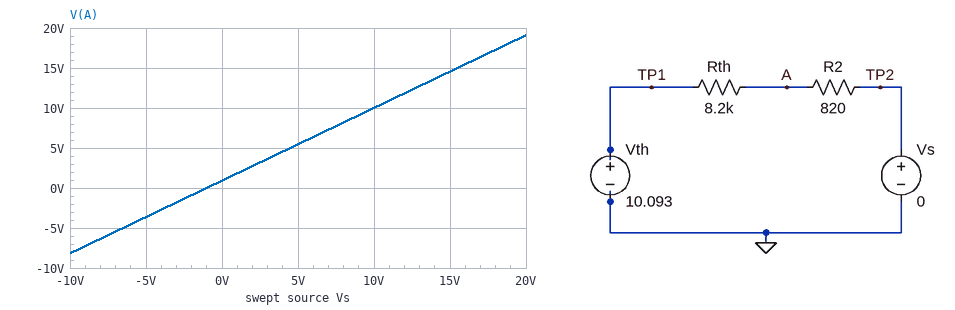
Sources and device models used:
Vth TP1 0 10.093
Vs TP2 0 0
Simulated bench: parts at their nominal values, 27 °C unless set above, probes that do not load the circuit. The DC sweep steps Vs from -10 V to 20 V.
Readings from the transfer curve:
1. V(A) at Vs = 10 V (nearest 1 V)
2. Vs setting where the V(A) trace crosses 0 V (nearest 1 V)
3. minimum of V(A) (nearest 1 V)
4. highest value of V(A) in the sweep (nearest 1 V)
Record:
10 V
-1 V
-8 V
19 V
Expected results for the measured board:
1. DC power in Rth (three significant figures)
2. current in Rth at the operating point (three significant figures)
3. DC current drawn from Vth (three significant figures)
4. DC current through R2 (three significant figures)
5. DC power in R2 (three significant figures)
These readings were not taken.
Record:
10.3 mW
1.12 mA
1.12 mA
1.12 mA
1.03 mW
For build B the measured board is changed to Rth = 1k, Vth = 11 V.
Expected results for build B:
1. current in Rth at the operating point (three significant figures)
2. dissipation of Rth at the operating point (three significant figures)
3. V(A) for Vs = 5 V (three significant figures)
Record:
6.04 mA
36.5 mW
7.70 V
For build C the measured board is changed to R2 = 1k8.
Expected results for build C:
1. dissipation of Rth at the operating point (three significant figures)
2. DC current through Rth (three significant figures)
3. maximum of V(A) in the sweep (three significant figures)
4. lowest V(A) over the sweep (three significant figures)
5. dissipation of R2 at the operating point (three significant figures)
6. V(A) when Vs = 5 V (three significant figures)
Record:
8.35 mW
1.01 mA
18.2 V
-6.38 V
1.83 mW
5.92 V
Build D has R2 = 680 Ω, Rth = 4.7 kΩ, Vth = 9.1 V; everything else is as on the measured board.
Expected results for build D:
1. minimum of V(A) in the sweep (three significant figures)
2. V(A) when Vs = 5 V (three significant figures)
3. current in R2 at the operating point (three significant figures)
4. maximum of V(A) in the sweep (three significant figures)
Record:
-7.59 V
5.52 V
1.69 mA
18.6 V
